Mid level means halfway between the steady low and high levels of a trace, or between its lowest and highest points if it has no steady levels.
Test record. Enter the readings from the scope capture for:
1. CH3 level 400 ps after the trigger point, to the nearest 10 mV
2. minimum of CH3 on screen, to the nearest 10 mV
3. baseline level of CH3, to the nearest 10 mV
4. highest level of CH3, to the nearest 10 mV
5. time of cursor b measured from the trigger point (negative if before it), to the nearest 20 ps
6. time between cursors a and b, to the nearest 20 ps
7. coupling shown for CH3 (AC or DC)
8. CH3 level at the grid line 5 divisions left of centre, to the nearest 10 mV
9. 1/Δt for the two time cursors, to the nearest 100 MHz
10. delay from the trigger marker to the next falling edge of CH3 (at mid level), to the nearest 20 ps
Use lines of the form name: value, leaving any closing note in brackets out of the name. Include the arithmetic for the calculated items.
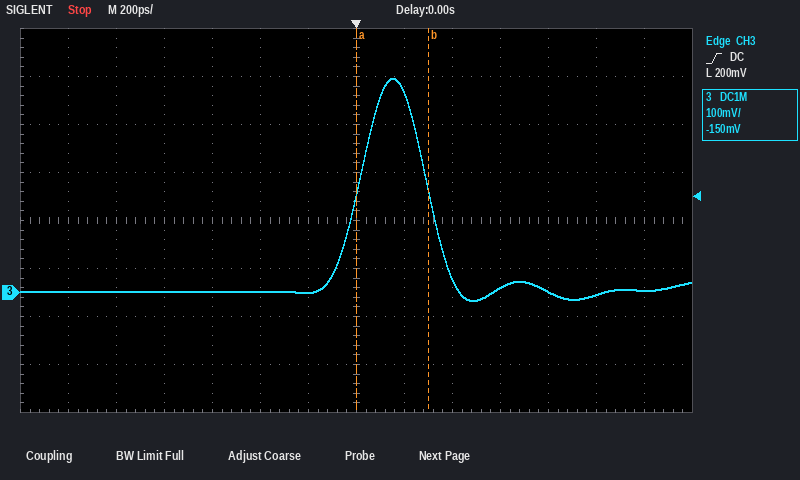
CH3 level 400 ps after the trigger point, to the nearest 10 mV: 30 mV
minimum of CH3 on screen, to the nearest 10 mV: -20 mV
baseline level of CH3, to the nearest 10 mV: 0 mV
highest level of CH3, to the nearest 10 mV: 450 mV
time of cursor b measured from the trigger point (negative if before it), to the nearest 20 ps: +300 ps
time between cursors a and b, to the nearest 20 ps: 300 ps
coupling shown for CH3: DC
CH3 level at the grid line 5 divisions left of centre, to the nearest 10 mV: 0 mV
1/Δt for the two time cursors, to the nearest 100 MHz: 1 / 300 ps ≈ 3.3 GHz
delay from the trigger marker to the next falling edge of CH3 (at mid level), to the nearest 20 ps: 300 ps
